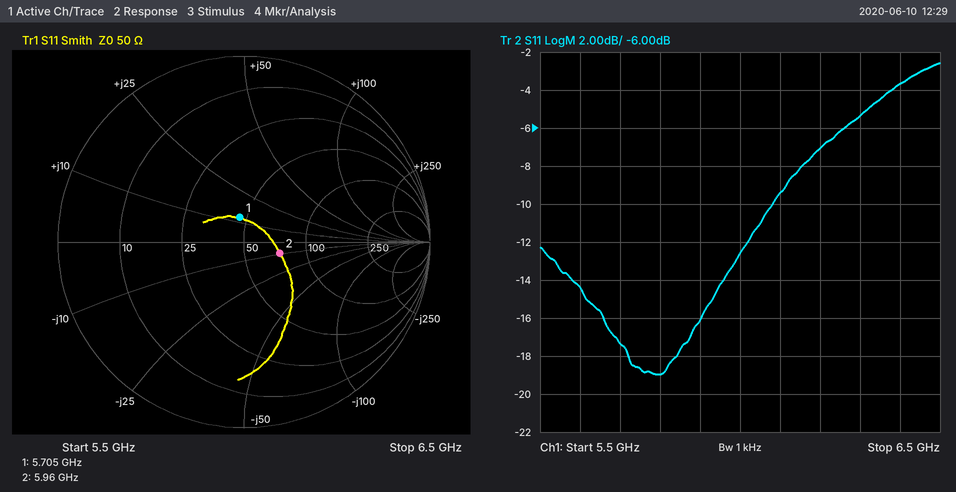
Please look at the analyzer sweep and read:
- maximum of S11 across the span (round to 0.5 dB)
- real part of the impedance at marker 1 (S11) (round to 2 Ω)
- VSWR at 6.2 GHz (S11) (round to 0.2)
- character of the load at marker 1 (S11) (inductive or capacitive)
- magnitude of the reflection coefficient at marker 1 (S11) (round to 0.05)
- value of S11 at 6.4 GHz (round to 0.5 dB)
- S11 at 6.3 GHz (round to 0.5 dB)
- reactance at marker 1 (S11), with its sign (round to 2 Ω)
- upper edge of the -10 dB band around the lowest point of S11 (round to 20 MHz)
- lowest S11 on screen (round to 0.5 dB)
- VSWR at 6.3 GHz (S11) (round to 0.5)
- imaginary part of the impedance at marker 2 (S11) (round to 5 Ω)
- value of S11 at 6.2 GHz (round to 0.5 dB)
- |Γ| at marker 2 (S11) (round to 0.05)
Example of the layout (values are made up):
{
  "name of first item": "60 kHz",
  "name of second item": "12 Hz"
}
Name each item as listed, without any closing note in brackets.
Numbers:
{
  "maximum of S11 across the span": "-2.5 dB",
  "real part of the impedance at marker 1 (S11)": "46 Ω",
  "VSWR at 6.2 GHz (S11)": "2.6",
  "character of the load at marker 1 (S11)": "inductive",
  "magnitude of the reflection coefficient at marker 1 (S11)": "0.15",
  "value of S11 at 6.4 GHz": "-3.5 dB",
  "S11 at 6.3 GHz": "-5.5 dB",
  "reactance at marker 1 (S11), with its sign": "+12 Ω",
  "upper edge of the -10 dB band around the lowest point of S11": "6.08 GHz",
  "lowest S11 on screen": "-19.0 dB",
  "VSWR at 6.3 GHz (S11)": "3.5",
  "imaginary part of the impedance at marker 2 (S11)": "-10 Ω",
  "value of S11 at 6.2 GHz": "-7.0 dB",
  "|Γ| at marker 2 (S11)": "0.20"
}
